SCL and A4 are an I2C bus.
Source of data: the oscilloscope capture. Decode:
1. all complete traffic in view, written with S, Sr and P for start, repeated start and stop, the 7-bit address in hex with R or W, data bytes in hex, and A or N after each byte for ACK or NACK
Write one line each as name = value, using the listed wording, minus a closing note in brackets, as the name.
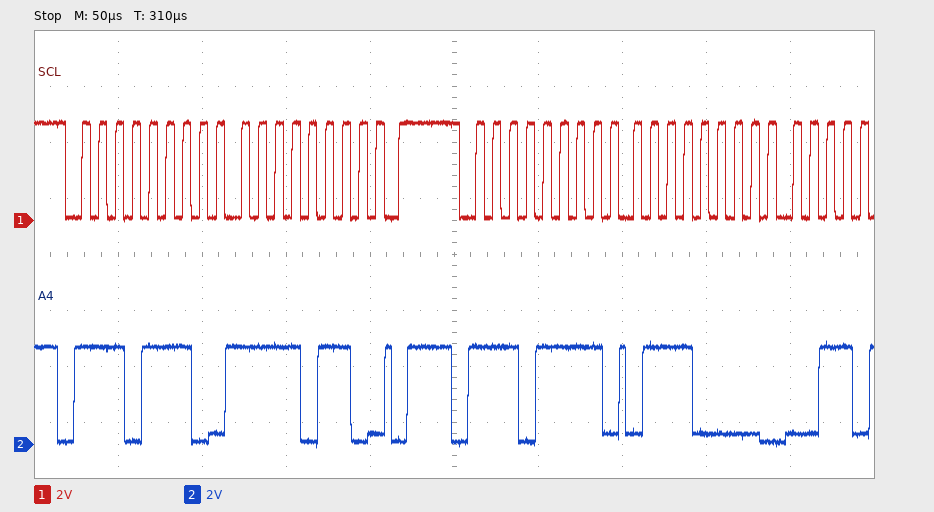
all complete traffic in view, written with S, Sr and P for start, repeated start and stop, the 7-bit address in hex with R or W, data bytes in hex, and A or N after each byte for ACK or NACK = S 77W A F6 A P S 77R A 70 A
